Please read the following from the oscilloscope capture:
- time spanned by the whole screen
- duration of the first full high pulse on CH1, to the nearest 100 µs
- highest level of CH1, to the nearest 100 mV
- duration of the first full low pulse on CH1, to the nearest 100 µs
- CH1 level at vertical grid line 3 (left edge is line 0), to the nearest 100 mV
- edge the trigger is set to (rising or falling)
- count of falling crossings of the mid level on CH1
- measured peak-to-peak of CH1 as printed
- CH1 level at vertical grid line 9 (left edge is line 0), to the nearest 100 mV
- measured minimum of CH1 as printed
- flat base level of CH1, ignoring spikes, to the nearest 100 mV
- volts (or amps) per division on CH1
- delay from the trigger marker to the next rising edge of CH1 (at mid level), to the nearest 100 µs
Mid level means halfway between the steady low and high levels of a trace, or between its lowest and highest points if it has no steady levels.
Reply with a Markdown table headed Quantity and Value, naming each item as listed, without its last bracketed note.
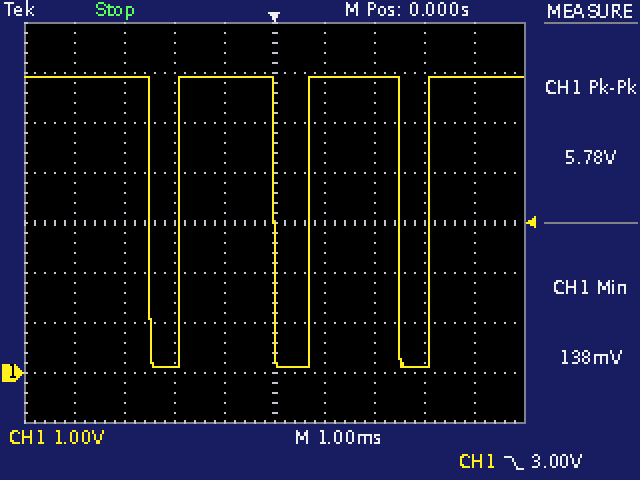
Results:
| Quantity | Value |
|---|---|
| time spanned by the whole screen | 10 ms |
| duration of the first full high pulse on CH1, to the nearest 100 µs | 1.9 ms |
| highest level of CH1, to the nearest 100 mV | 5.9 V |
| duration of the first full low pulse on CH1, to the nearest 100 µs | 600 µs |
| CH1 level at vertical grid line 3 (left edge is line 0), to the nearest 100 mV | 100 mV |
| edge the trigger is set to | falling |
| count of falling crossings of the mid level on CH1 | 3 |
| measured peak-to-peak of CH1 as printed | 5.78 V |
| CH1 level at vertical grid line 9 (left edge is line 0), to the nearest 100 mV | 5.9 V |
| measured minimum of CH1 as printed | 138 mV |
| flat base level of CH1, ignoring spikes, to the nearest 100 mV | 100 mV |
| volts (or amps) per division on CH1 | 1 V |
| delay from the trigger marker to the next rising edge of CH1 (at mid level), to the nearest 100 µs | 700 µs |
